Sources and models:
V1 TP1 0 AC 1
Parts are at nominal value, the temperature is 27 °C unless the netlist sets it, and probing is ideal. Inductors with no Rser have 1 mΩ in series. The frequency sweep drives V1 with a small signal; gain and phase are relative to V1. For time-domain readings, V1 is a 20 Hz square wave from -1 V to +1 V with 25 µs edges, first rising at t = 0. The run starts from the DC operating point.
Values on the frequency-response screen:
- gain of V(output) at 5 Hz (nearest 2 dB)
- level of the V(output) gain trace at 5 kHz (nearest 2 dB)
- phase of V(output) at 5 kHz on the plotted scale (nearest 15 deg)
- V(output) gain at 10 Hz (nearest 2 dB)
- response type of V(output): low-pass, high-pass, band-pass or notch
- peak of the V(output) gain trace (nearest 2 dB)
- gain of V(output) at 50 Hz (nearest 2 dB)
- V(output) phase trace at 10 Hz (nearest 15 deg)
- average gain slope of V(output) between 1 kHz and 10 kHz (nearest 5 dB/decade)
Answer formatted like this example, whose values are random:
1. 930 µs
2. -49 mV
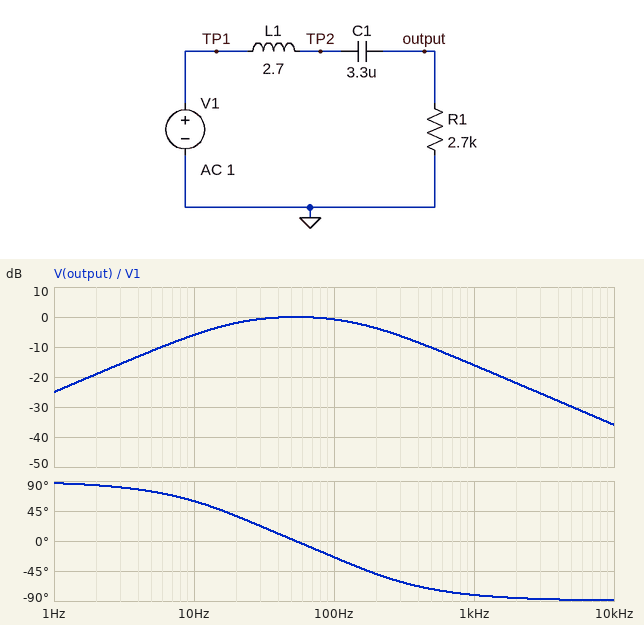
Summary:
1. -12 dB
2. -30 dB
3. -90 deg
4. -6 dB
5. band-pass
6. 0 dB
7. 0 dB
8. 60 deg
9. -20 dB/decade
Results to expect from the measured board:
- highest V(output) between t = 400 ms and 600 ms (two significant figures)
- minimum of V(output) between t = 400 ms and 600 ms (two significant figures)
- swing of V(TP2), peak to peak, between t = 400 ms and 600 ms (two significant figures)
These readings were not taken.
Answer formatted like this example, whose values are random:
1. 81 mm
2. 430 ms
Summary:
1. 1.6 V
2. -1.6 V
3. 2.3 V
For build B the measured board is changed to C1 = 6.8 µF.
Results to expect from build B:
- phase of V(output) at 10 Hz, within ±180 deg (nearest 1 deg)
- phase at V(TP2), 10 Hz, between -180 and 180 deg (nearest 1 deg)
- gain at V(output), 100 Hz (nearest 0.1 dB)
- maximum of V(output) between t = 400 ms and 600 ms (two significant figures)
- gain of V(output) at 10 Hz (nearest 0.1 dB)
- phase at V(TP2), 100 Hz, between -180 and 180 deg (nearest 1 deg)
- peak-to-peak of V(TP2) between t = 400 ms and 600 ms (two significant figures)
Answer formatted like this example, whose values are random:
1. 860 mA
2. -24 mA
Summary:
1. 39 deg
2. -2 deg
3. -1.1 dB
4. 1.4 V
5. -2.2 dB
6. -33 deg
7. 2.1 V
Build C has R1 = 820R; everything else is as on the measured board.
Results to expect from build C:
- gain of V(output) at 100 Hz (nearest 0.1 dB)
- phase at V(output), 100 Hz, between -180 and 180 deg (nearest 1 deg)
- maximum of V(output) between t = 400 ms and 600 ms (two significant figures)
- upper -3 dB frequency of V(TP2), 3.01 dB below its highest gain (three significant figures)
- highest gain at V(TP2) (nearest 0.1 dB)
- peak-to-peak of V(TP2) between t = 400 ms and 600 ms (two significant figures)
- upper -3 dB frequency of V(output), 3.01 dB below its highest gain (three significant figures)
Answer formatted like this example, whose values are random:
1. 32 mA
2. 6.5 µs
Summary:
1. -5.0 dB
2. -56 deg
3. 1.0 V
4. 71.1 Hz
5. 3.8 dB
6. 3.3 V
7. 82.7 Hz
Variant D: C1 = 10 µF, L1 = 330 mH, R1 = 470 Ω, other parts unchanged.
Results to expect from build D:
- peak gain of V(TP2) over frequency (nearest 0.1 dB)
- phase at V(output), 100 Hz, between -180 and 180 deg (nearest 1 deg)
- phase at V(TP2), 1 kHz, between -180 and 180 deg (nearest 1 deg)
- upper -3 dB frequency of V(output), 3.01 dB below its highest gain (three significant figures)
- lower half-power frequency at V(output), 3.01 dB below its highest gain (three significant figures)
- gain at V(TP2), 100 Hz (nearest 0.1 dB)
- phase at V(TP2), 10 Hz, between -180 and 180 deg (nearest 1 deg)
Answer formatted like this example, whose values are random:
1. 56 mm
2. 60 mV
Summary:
1. 0.8 dB
2. -6 deg
3. -79 deg
4. 257 Hz
5. 29.9 Hz
6. 0.4 dB
7. 0 deg
